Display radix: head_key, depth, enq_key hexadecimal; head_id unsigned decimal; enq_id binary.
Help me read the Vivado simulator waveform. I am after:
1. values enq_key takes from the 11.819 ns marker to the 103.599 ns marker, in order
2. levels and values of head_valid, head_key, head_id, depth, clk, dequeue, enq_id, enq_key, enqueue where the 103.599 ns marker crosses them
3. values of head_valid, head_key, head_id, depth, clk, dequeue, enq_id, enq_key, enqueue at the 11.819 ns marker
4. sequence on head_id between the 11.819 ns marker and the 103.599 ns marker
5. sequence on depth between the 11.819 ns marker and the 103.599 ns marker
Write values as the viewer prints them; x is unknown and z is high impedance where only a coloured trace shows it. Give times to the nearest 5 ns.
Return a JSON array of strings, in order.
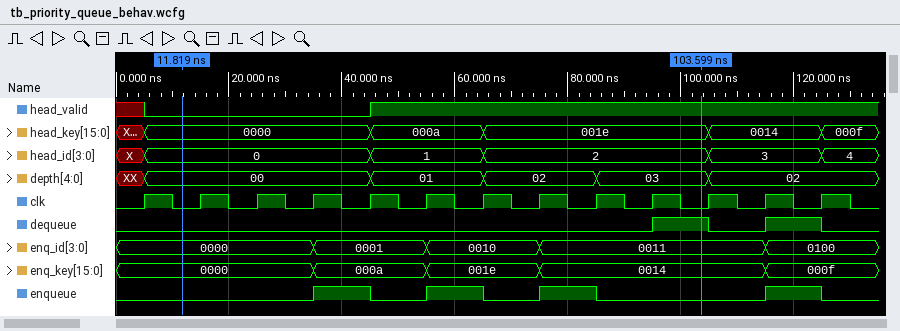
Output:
["0000, 000a, 001e, 0014", "head_valid=1, head_key=001e, head_id=2, depth=03, clk=0, dequeue=1, enq_id=0011, enq_key=0014, enqueue=0", "head_valid=0, head_key=0000, head_id=0, depth=00, clk=0, dequeue=0, enq_id=0000, enq_key=0000, enqueue=0", "0, 1, 2", "00, 01, 02, 03"]
